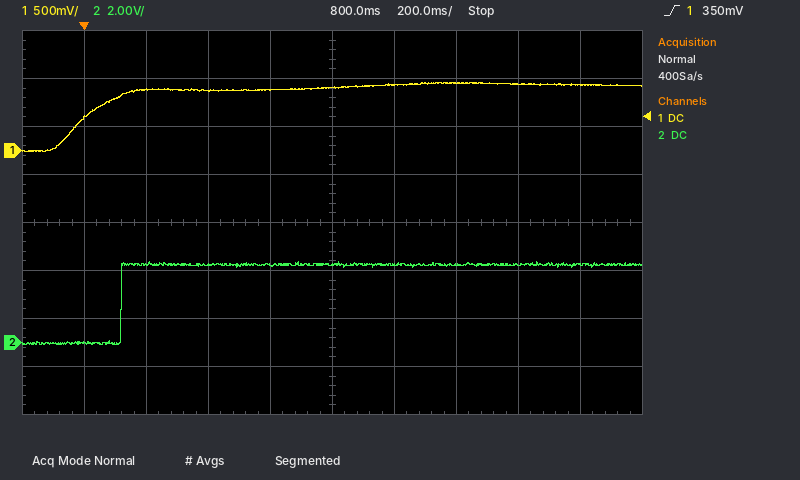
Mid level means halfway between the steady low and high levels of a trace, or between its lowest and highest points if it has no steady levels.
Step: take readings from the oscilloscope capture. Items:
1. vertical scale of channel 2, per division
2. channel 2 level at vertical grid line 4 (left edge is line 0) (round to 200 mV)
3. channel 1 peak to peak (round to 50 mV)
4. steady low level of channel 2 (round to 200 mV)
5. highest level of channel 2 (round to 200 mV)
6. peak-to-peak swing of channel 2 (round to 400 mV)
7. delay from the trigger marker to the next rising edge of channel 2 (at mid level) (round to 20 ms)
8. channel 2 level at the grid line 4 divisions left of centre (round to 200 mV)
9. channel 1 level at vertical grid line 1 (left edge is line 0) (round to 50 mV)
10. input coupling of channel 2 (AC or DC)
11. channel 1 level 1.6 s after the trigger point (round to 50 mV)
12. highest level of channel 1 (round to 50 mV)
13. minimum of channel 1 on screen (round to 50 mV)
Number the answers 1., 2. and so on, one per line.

1. 2 V
2. 3.2 V
3. 700 mV
4. 0.0 V
5. 3.4 V
6. 3.6 V
7. 120 ms
8. 0.0 V
9. 350 mV
10. DC
11. 700 mV
12. 700 mV
13. 0 mV
